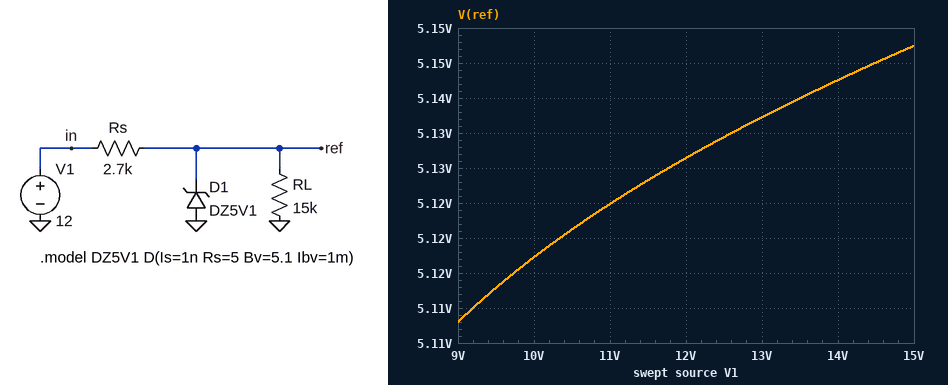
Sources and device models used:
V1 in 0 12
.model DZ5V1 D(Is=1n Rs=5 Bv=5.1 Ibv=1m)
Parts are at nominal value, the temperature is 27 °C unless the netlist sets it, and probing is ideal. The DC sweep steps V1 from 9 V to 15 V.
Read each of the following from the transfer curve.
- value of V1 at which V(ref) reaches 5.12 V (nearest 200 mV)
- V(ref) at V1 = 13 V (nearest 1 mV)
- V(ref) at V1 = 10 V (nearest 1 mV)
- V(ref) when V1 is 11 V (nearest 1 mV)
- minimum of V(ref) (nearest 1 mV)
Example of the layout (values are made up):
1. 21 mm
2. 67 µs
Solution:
1. 10.4 V
2. 5.137 V
3. 5.117 V
4. 5.125 V
5. 5.108 V
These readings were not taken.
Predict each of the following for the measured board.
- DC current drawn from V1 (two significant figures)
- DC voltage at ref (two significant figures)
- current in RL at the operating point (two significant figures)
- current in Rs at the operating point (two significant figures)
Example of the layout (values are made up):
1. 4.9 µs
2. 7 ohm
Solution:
1. 2.5 mA
2. 5.1 V
3. 340 µA
4. 2.5 mA
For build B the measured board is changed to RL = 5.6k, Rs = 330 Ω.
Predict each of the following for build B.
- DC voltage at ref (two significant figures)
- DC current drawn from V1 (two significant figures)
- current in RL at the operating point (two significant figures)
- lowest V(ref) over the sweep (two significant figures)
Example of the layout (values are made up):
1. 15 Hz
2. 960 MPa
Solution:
1. 5.3 V
2. 20 mA
3. 940 µA
4. 5.2 V
